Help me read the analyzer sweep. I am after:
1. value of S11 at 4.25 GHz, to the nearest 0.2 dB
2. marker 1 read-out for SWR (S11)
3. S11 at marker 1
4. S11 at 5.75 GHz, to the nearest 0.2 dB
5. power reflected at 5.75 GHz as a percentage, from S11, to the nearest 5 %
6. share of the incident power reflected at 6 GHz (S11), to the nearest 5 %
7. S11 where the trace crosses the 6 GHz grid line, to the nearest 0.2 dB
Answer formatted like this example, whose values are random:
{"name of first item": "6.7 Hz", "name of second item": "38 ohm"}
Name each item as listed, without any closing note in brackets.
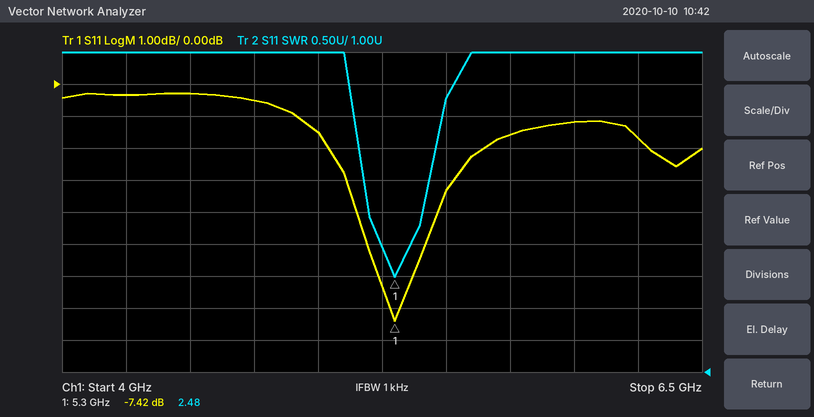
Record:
{"value of S11 at 4.25 GHz, to the nearest 0.2 dB": "-0.4 dB", "marker 1 read-out for SWR": "2.48", "S11 at marker 1": "-7.42 dB", "S11 at 5.75 GHz, to the nearest 0.2 dB": "-1.6 dB", "power reflected at 5.75 GHz as a percentage, from S11, to the nearest 5 %": "70 %", "share of the incident power reflected at 6 GHz (S11), to the nearest 5 %": "75 %", "S11 where the trace crosses the 6 GHz grid line, to the nearest 0.2 dB": "-1.2 dB"}
